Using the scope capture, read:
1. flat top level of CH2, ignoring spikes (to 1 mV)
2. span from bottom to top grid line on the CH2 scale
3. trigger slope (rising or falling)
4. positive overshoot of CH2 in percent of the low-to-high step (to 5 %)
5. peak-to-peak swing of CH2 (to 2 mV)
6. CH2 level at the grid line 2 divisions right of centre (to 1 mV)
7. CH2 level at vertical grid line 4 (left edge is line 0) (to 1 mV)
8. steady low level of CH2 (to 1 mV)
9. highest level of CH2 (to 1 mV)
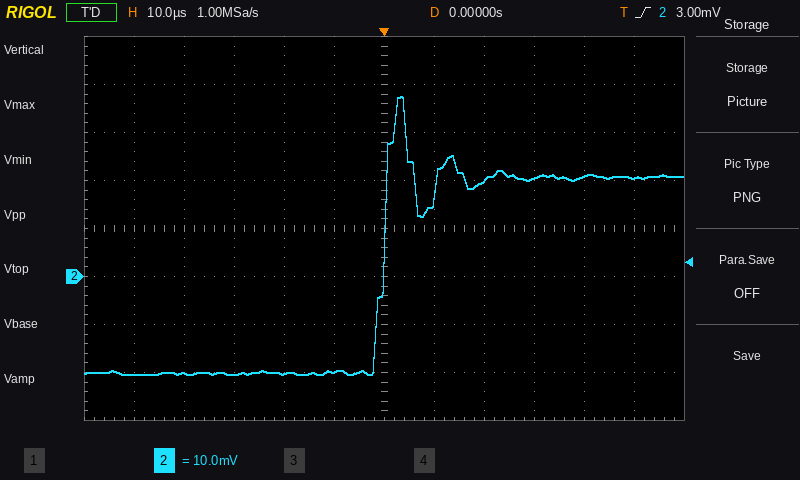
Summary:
21 mV
80 mV
rising
40 %
58 mV
20 mV
-20 mV
-20 mV
38 mV
